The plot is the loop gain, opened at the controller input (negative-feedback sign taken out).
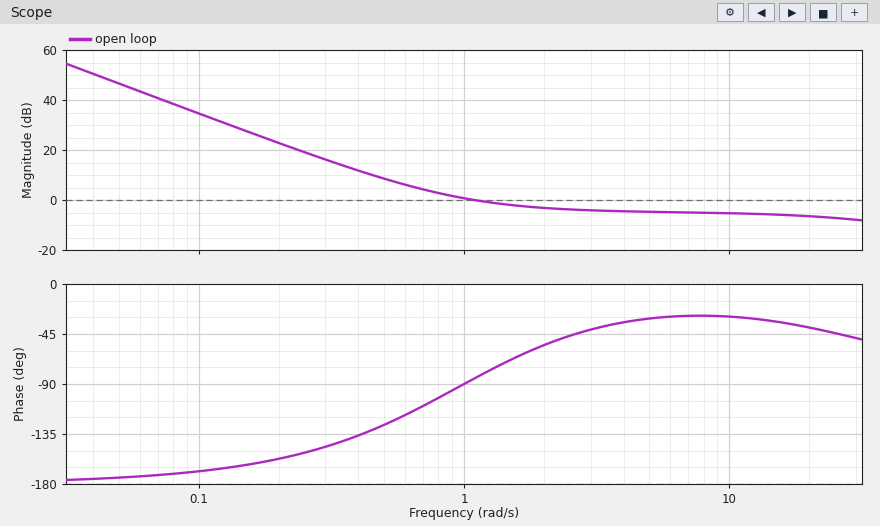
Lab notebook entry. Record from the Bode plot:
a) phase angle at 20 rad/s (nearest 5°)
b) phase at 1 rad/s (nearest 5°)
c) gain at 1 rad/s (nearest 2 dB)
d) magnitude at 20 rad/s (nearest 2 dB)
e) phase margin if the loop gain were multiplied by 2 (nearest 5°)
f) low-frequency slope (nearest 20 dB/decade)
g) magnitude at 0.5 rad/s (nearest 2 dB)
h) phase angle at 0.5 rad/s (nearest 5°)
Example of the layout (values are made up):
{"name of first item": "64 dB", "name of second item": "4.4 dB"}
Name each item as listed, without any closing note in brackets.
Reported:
{"phase angle at 20 rad/s": "-40°", "phase at 1 rad/s": "-90°", "gain at 1 rad/s": "0 dB", "magnitude at 20 rad/s": "-6 dB", "phase margin if the loop gain were multiplied by 2": "145°", "low-frequency slope": "-40 dB/decade", "magnitude at 0.5 rad/s": "8 dB", "phase angle at 0.5 rad/s": "-125°"}
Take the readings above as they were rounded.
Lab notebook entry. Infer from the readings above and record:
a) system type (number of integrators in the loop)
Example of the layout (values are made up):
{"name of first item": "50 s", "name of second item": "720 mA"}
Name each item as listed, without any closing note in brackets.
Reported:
{"system type": "2"}
